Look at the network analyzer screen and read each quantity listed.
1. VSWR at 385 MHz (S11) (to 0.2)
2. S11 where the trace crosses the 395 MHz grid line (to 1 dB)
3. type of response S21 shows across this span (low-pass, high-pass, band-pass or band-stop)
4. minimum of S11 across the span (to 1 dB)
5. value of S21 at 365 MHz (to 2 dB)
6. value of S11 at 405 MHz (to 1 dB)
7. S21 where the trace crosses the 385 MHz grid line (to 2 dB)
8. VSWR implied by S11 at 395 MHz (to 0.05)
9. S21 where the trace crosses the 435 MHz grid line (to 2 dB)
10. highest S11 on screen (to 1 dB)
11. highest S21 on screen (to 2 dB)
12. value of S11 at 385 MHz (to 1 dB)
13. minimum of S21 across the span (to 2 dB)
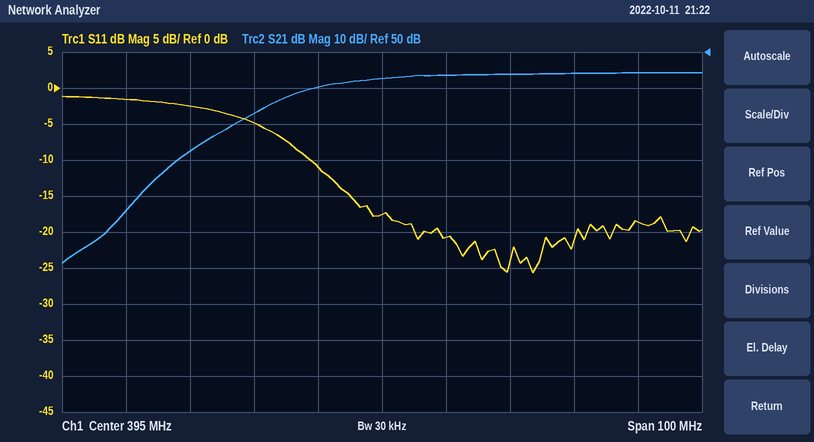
1.8
-18 dB
high-pass
-26 dB
22 dB
-21 dB
40 dB
1.30
44 dB
-1 dB
44 dB
-11 dB
-8 dB
